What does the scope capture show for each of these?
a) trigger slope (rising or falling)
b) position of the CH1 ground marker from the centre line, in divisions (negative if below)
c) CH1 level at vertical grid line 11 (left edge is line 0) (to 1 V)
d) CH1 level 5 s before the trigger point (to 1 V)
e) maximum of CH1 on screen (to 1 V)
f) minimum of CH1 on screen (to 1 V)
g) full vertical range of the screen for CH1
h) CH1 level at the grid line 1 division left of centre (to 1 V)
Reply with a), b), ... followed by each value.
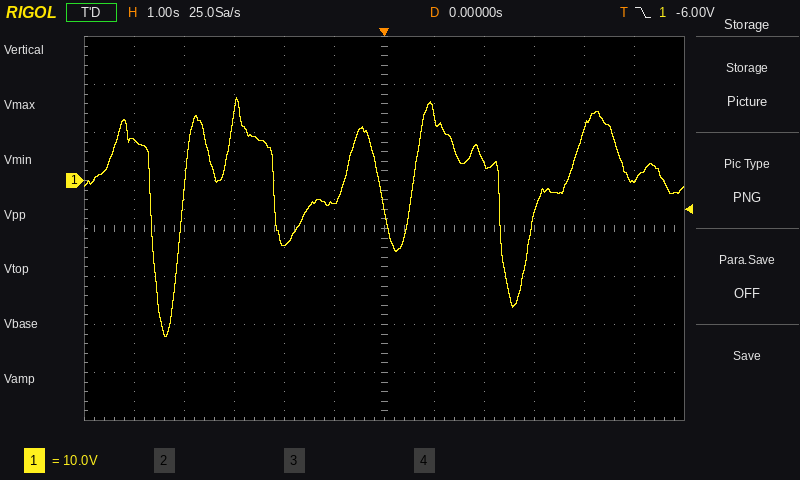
a) falling
b) +1.0 div
c) 0 V
d) 8 V
e) 17 V
f) -32 V
g) 80 V
h) -5 V
